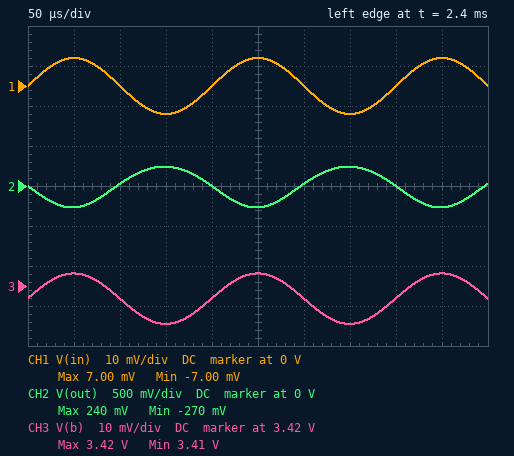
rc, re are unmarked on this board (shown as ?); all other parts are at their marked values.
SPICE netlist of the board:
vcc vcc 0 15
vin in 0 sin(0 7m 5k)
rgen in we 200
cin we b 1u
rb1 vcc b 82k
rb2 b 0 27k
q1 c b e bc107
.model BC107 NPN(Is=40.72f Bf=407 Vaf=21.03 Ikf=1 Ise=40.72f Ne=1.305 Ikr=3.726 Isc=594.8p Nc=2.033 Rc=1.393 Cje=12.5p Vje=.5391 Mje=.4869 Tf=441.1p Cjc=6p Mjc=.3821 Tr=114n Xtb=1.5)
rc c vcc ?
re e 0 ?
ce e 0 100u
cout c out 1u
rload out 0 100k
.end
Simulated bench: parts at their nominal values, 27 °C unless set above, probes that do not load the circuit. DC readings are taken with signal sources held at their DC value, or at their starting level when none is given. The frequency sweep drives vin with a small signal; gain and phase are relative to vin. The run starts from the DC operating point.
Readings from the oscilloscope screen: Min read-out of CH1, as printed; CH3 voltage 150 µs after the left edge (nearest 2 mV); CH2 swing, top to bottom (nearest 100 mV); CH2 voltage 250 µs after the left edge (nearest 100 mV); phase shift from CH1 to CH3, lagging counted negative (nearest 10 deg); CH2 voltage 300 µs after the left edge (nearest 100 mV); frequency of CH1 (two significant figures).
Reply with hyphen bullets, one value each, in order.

- -7.00 mV
- 3.410 V
- 500 mV
- -300 mV
- 0 deg
- 0 V
- 5.0 kHz
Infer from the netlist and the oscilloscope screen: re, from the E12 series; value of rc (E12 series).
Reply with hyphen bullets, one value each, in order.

- 680 Ω
- 270 Ω
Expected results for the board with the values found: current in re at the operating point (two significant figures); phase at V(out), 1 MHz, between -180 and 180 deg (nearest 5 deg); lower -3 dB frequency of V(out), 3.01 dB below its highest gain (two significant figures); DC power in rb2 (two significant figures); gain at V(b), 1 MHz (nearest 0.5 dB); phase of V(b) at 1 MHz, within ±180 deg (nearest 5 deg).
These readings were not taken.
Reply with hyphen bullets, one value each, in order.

- 4.1 mA
- 170 deg
- 290 Hz
- 430 µW
- -1.0 dB
- -10 deg
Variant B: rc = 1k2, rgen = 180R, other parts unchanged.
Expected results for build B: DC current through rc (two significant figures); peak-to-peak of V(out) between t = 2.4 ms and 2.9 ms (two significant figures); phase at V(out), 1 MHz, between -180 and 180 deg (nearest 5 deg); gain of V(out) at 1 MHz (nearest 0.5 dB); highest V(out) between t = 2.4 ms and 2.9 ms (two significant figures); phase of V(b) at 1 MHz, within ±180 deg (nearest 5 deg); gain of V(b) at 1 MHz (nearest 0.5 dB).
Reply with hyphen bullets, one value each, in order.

- 4.0 mA
- 2.0 V
- 155 deg
- 42.0 dB
- 950 mV
- -25 deg
- -2.0 dB
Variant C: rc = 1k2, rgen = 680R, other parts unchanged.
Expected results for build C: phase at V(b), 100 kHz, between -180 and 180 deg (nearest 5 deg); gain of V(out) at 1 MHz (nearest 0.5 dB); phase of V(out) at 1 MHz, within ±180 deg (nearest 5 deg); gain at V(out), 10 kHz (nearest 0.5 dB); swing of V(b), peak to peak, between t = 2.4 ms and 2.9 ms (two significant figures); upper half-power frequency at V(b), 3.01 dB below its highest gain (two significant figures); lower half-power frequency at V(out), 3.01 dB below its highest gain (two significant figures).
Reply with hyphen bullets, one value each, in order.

- -10 deg
- 36.0 dB
- 125 deg
- 41.0 dB
- 10 mV
- 680 kHz
- 220 Hz
